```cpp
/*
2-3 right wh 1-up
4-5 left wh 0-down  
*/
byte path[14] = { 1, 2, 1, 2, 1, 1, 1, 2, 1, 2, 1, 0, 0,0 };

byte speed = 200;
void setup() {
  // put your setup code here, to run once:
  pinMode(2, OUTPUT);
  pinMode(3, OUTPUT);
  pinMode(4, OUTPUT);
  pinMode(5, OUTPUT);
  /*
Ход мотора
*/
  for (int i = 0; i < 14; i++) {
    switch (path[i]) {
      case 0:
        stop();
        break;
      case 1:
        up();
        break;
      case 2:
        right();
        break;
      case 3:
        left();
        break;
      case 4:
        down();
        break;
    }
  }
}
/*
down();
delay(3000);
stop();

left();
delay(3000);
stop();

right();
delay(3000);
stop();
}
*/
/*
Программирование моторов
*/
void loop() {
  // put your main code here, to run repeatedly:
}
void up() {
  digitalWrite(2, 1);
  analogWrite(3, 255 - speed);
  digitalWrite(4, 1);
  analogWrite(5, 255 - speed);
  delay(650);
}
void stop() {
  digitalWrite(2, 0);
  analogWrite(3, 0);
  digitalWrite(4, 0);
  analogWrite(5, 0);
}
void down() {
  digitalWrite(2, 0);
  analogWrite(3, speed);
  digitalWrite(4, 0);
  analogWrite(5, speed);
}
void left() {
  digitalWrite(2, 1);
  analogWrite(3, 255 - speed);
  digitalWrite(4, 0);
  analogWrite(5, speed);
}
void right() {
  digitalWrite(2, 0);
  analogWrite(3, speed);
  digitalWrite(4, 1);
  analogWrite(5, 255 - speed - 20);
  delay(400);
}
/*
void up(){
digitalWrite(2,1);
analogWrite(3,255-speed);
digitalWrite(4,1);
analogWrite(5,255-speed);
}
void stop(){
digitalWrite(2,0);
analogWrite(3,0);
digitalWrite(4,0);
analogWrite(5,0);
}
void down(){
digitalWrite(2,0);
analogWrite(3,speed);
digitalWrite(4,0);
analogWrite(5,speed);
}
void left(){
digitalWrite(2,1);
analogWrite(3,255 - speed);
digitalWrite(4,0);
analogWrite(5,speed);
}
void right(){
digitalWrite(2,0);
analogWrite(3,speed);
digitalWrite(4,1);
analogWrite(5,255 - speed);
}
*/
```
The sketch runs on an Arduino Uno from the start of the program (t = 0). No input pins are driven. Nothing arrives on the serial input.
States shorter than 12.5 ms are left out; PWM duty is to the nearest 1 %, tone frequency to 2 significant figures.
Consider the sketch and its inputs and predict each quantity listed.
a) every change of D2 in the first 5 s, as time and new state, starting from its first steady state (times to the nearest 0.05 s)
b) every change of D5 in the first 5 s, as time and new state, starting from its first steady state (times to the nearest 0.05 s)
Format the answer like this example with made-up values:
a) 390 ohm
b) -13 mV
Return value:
a) 0 s high; 0.65 s low; 1.05 s high; 1.7 s low; 2.1 s high; 4.05 s low; 4.45 s high
b) 0 s PWM 22 %; 0.65 s PWM 14 %; 1.05 s PWM 22 %; 1.7 s PWM 14 %; 2.1 s PWM 22 %; 4.05 s PWM 14 %; 4.45 s PWM 22 %
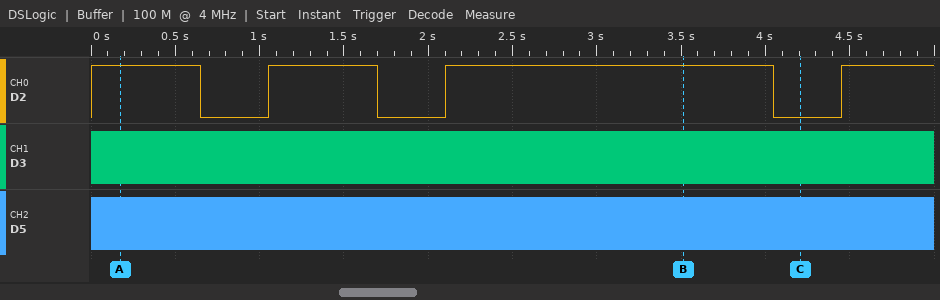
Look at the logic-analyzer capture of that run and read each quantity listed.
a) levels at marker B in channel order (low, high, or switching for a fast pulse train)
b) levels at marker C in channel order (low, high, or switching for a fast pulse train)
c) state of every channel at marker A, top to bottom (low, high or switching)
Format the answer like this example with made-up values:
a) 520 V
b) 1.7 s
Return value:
a) D2 high, D3 switching, D5 switching
b) D2 low, D3 switching, D5 switching
c) D2 high, D3 switching, D5 switching
